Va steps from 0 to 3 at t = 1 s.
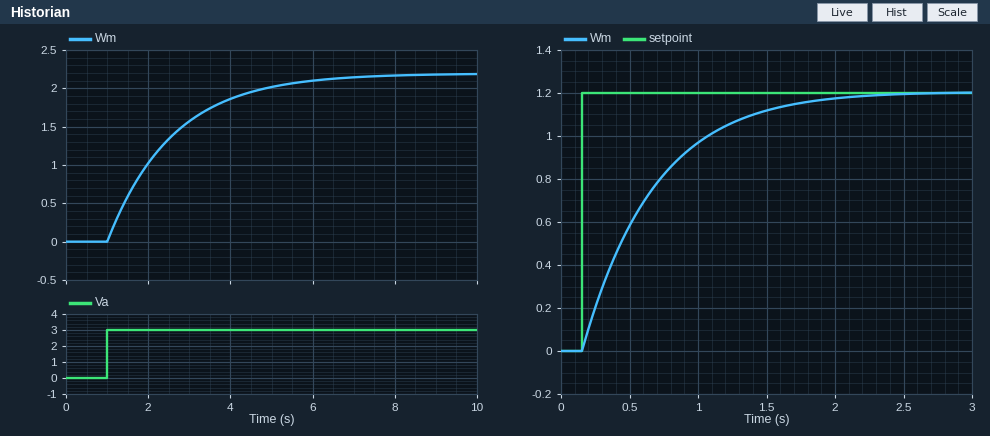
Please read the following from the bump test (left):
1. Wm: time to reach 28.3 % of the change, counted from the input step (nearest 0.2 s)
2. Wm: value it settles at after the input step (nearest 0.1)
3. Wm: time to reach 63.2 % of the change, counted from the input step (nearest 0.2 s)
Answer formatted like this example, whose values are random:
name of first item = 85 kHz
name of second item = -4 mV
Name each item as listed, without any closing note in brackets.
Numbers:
Wm: time to reach 28.3 % of the change, counted from the input step = 0.6 s
Wm: value it settles at after the input step = 2.2
Wm: time to reach 63.2 % of the change, counted from the input step = 1.6 s
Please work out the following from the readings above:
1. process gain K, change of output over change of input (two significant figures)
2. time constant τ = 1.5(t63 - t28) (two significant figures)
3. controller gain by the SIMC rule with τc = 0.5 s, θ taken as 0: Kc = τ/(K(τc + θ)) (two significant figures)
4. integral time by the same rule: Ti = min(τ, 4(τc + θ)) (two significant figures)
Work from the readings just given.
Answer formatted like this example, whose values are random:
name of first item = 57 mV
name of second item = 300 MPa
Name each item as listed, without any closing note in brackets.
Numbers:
process gain K, change of output over change of input = 0.73
time constant τ = 1.5(t63 - t28) = 1.5 s
controller gain by the SIMC rule with τc = 0.5 s, θ taken as 0: Kc = τ/(K(τc + θ)) = 4.1
integral time by the same rule: Ti = min(τ, 4(τc + θ)) = 1.5 s
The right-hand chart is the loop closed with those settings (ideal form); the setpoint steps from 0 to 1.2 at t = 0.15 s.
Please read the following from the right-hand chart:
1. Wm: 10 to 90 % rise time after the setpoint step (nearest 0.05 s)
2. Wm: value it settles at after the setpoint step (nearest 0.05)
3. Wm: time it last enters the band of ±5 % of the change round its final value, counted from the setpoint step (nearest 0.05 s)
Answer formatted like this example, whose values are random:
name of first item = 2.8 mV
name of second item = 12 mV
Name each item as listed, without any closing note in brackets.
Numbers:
Wm: 10 to 90 % rise time after the setpoint step = 1.10 s
Wm: value it settles at after the setpoint step = 1.20
Wm: time it last enters the band of ±5 % of the change round its final value, counted from the setpoint step = 1.50 s
